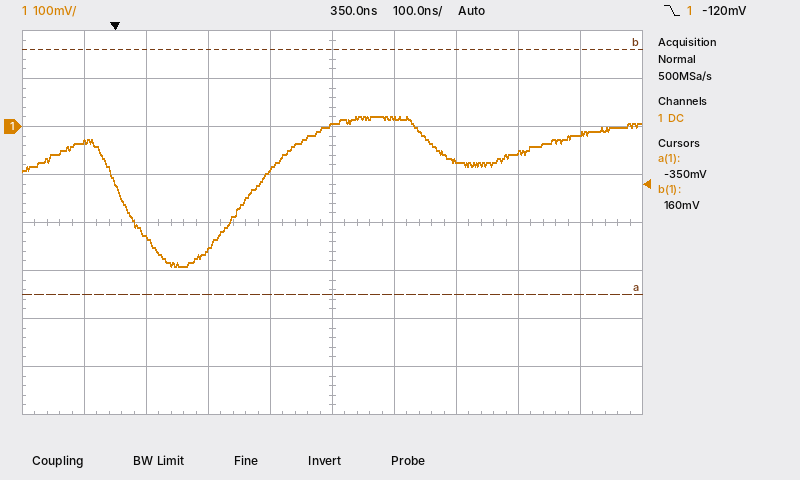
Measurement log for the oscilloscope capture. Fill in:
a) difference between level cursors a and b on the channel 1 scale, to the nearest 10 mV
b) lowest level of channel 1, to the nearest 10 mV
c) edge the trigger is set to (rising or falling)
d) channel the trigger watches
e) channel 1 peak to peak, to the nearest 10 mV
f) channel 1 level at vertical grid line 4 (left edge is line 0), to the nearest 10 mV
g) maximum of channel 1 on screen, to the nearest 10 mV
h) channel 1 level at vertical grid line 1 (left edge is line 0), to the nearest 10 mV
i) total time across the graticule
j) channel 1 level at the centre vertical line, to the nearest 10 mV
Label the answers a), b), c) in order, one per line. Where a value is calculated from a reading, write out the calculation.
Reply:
a) 510 mV
b) -290 mV
c) falling
d) channel 1
e) 20 mV − (-290 mV) = 310 mV
f) -90 mV
g) 20 mV
h) -30 mV
i) 1 µs
j) 0 mV
